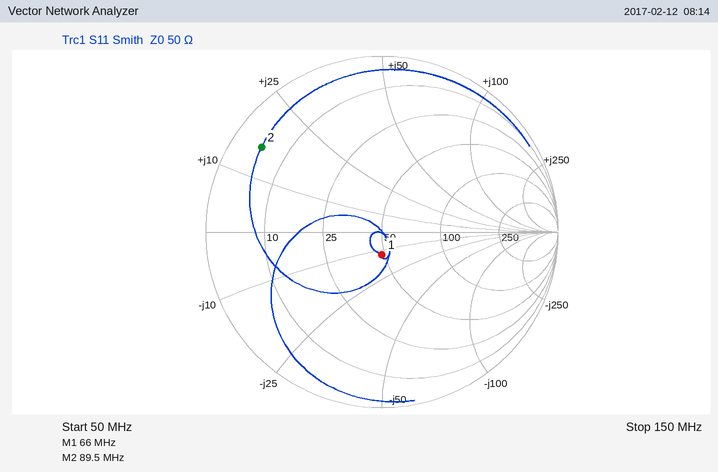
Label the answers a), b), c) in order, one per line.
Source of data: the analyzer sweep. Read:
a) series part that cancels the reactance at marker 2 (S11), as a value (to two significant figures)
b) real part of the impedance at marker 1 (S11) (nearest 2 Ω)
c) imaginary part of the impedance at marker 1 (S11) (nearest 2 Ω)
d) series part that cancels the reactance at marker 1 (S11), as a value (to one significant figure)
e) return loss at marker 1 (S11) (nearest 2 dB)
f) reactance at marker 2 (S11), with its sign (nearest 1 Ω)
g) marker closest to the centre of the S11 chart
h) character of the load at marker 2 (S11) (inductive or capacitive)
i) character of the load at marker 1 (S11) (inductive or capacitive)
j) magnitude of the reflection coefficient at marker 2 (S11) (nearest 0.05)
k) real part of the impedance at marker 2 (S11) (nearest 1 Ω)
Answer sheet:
a) 110 pF
b) 48 Ω
c) -12 Ω
d) 30 nH
e) 18 dB
f) +16 Ω
g) marker 1
h) inductive
i) capacitive
j) 0.85
k) 5 Ω
